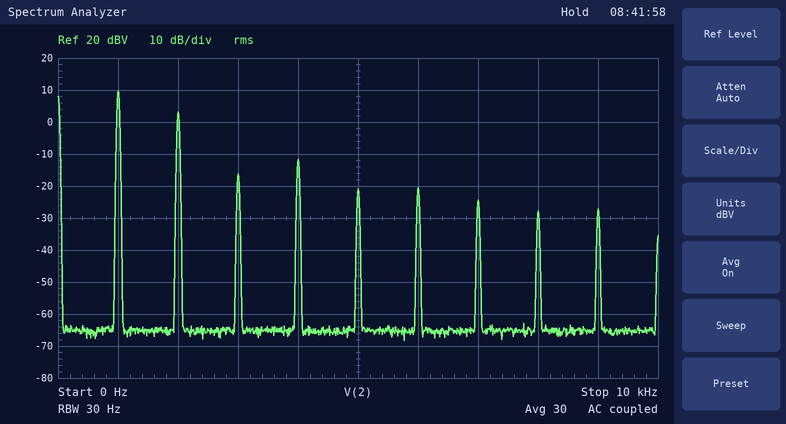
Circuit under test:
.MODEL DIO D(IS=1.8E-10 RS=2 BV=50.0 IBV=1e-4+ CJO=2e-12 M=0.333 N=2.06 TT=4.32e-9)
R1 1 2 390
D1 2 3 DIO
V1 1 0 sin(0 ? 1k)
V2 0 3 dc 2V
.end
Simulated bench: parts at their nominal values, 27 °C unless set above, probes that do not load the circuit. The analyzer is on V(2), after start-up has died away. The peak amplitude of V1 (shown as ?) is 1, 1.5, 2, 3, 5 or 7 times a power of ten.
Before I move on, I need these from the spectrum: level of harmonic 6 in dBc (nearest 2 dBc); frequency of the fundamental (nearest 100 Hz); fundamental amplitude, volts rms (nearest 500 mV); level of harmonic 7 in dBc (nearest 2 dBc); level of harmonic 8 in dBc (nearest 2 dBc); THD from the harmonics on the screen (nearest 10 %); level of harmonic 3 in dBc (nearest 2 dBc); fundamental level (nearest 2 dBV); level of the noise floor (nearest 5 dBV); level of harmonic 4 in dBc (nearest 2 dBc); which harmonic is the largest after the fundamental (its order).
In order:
-30 dBc
1.0 kHz
3.0 V
-34 dBc
-38 dBc
50 %
-26 dBc
10 dBV
-65 dBV
-22 dBc
2
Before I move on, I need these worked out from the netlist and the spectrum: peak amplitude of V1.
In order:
10 V
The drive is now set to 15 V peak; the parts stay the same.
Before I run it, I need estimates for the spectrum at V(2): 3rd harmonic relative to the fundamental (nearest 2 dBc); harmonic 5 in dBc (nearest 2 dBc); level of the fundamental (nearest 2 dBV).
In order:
-30 dBc
-34 dBc
14 dBV
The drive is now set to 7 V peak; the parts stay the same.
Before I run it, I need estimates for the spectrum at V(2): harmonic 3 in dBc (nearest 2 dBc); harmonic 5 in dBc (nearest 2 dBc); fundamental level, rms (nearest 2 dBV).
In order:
-22 dBc
-28 dBc
6 dBV
